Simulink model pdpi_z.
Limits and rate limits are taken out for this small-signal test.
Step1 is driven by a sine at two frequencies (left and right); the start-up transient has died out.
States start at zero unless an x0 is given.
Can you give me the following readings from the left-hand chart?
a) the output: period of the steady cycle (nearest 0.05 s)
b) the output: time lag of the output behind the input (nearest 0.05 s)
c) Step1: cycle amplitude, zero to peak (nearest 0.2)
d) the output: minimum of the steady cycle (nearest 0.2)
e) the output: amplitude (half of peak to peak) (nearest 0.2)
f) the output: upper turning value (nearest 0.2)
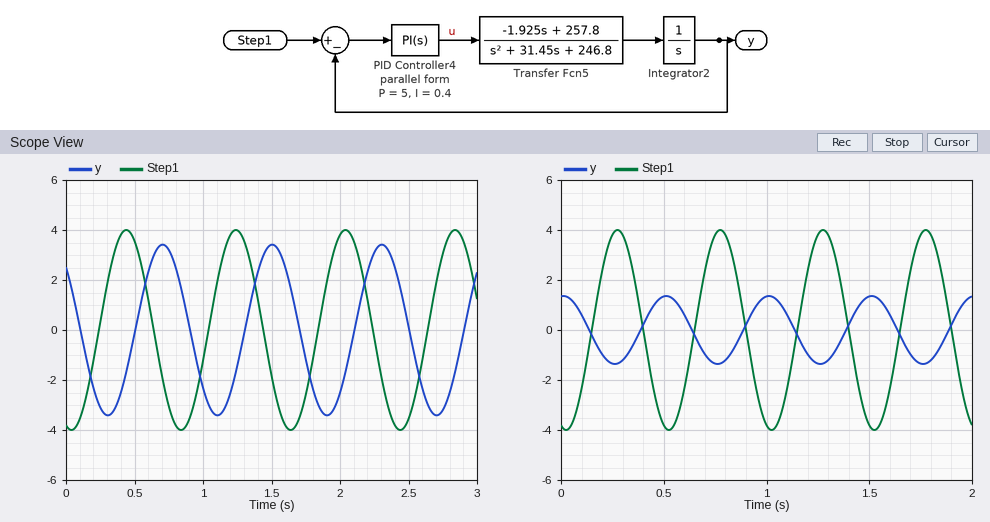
0.80 s
0.25 s
4.0
-3.4
3.4
3.4
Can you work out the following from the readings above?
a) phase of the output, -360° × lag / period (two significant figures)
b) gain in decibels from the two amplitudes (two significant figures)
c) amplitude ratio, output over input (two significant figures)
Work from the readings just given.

-110°
-1.4 dB
0.85
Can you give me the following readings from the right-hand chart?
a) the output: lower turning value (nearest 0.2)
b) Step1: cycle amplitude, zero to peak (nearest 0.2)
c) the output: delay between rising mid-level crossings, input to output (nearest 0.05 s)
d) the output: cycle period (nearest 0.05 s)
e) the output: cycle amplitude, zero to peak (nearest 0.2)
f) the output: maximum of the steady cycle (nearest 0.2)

-1.4
4.0
0.25 s
0.50 s
1.4
1.4
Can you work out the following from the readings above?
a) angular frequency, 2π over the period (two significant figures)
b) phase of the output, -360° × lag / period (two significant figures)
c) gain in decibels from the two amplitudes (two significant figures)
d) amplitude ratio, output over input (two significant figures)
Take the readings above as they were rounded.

13 rad/s
-180°
-9.1 dB
0.35
